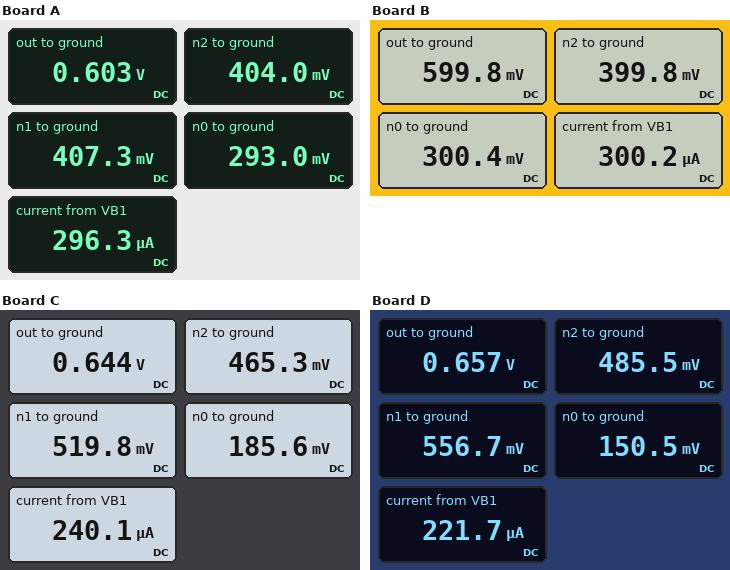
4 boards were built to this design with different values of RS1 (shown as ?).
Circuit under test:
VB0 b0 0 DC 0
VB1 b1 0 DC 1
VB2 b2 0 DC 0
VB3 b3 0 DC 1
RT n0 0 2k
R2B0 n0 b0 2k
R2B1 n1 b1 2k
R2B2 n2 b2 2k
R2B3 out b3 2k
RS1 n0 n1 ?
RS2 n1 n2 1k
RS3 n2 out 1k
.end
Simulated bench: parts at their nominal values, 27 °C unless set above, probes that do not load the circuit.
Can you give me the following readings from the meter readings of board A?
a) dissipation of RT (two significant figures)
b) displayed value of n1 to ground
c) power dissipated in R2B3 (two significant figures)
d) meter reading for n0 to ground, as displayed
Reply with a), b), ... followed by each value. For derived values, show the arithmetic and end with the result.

a) (293 mV)^2 / 2 kΩ = 43 µW
b) 407.3 mV
c) (1 V - 603 mV)^2 / 2 kΩ = 79 µW
d) 293.0 mV
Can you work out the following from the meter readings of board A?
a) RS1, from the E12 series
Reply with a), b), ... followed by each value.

a) 390 Ω
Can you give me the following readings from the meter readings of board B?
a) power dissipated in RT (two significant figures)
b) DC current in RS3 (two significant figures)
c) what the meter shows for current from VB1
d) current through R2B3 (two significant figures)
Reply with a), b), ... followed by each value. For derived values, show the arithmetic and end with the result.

a) (300.4 mV)^2 / 2 kΩ = 45 µW
b) (599.8 mV - 399.8 mV) / 1 kΩ = 200 µA
c) 300.2 µA
d) (1 V - 599.8 mV) / 2 kΩ = 200 µA
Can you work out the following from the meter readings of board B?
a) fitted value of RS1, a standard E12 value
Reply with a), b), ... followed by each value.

a) 330 Ω
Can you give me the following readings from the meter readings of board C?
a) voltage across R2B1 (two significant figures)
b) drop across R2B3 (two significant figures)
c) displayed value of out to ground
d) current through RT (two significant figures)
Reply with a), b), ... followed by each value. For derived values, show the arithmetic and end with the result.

a) 1 V - 519.8 mV = 480 mV
b) 1 V - 644 mV = 360 mV
c) 0.644 V
d) (185.6 mV) / 2 kΩ = 93 µA
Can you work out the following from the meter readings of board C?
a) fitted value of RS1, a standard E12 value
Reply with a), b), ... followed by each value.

a) 1.8 kΩ
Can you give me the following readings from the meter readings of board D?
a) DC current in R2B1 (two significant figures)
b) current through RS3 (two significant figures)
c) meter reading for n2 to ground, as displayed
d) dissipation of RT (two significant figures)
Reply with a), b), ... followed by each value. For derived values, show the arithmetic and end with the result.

a) (1 V - 556.7 mV) / 2 kΩ = 220 µA
b) (657 mV - 485.5 mV) / 1 kΩ = 170 µA
c) 485.5 mV
d) (150.5 mV)^2 / 2 kΩ = 11 µW
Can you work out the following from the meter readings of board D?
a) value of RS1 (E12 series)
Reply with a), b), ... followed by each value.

a) 2.7 kΩ
